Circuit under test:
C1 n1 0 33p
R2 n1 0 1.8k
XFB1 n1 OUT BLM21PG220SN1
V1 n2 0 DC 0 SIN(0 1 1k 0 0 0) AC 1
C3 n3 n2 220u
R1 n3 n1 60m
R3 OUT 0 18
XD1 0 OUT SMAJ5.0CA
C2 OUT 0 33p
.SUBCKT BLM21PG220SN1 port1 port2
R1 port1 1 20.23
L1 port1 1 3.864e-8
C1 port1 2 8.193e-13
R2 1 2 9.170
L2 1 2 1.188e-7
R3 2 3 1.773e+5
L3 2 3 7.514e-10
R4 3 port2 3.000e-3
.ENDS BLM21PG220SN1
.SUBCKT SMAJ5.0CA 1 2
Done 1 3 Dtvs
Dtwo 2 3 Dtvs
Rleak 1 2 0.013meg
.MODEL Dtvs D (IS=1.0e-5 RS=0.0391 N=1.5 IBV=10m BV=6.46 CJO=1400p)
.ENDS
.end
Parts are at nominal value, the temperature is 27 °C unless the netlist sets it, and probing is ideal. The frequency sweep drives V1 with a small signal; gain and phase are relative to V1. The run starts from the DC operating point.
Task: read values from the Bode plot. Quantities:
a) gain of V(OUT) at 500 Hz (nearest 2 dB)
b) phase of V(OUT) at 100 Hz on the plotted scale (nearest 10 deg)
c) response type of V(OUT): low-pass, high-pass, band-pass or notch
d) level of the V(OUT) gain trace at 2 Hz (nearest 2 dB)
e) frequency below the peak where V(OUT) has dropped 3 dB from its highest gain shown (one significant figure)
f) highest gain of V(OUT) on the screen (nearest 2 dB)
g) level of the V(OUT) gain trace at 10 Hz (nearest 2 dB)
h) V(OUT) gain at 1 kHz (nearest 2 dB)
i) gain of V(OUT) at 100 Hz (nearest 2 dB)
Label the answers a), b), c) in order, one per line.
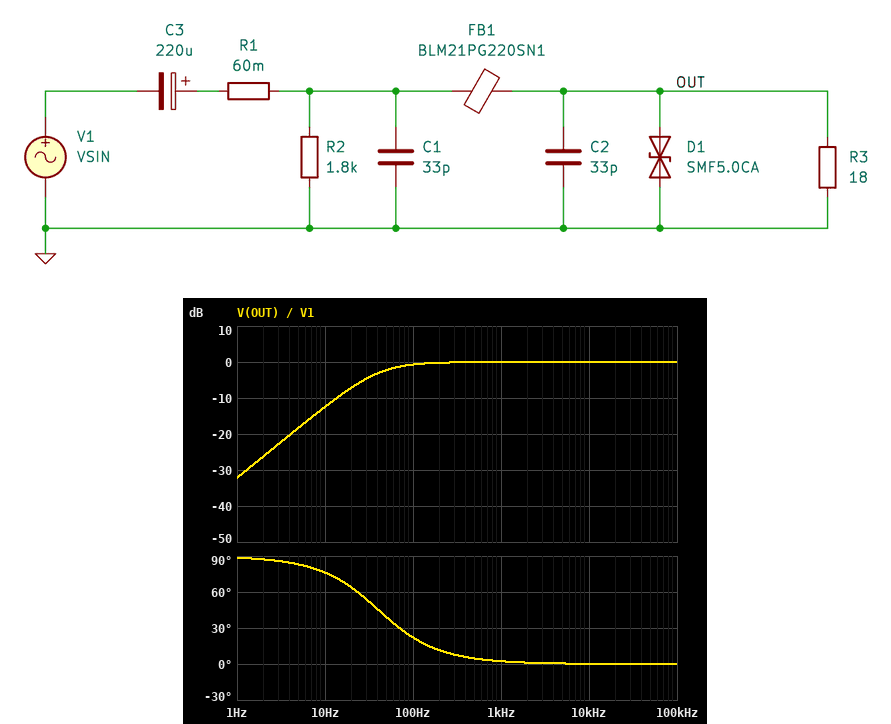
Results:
a) 0 dB
b) 20 deg
c) high-pass
d) -26 dB
e) 40 Hz
f) 0 dB
g) -12 dB
h) 0 dB
i) 0 dB
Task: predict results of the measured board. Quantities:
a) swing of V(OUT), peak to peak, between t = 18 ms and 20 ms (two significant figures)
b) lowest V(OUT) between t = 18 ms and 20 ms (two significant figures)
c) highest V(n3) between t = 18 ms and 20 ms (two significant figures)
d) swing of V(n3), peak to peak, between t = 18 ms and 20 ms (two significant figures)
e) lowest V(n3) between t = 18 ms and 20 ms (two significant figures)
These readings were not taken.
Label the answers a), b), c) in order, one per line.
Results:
a) 2.0 V
b) -1.0 V
c) 1.0 V
d) 2.0 V
e) -1.0 V
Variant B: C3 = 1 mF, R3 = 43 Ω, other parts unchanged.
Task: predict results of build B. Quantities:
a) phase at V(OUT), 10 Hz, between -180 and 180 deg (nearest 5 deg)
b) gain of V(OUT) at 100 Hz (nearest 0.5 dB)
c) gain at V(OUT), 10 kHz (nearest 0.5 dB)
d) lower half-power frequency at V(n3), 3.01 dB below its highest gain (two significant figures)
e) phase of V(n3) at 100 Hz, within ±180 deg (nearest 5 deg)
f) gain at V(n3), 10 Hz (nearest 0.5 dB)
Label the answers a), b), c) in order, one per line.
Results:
a) 20 deg
b) 0 dB
c) 0 dB
d) 3.8 Hz
e) 0 deg
f) -0.5 dB
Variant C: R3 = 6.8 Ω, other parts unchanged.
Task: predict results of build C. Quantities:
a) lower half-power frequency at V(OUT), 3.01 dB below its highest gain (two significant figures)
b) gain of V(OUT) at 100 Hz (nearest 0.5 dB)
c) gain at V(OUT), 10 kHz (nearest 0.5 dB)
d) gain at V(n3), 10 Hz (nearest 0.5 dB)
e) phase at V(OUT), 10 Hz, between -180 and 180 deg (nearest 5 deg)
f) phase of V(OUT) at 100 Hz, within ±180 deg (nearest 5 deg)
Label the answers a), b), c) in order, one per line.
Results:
a) 110 Hz
b) -3.5 dB
c) 0 dB
d) -20.5 dB
e) 85 deg
f) 45 deg
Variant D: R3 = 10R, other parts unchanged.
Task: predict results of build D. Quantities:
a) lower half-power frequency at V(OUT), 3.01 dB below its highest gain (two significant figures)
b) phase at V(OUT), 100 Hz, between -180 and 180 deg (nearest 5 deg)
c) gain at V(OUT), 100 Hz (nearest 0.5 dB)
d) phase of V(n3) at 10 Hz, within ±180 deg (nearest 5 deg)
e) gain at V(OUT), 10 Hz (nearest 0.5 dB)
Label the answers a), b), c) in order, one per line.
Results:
a) 72 Hz
b) 35 deg
c) -2.0 dB
d) 80 deg
e) -17.5 dB
